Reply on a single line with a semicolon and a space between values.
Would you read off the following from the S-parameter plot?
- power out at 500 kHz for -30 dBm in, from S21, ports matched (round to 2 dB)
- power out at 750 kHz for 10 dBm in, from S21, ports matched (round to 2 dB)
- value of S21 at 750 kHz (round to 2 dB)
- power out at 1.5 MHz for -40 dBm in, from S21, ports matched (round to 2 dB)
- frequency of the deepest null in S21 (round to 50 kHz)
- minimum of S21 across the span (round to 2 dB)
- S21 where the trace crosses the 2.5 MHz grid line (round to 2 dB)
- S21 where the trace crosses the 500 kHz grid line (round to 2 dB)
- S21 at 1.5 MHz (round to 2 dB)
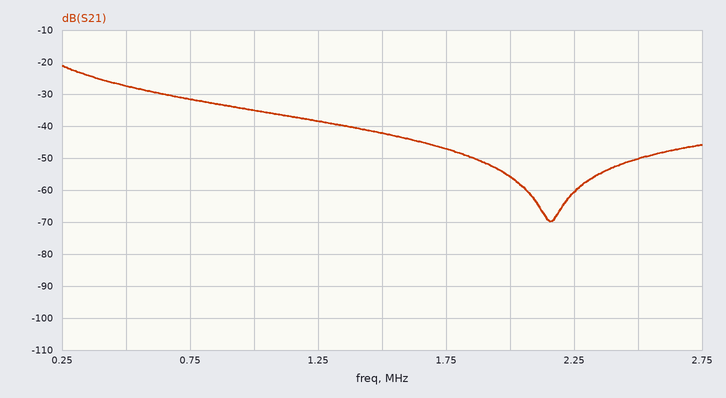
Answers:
-58 dBm; -22 dBm; -32 dB; -82 dBm; 2.15 MHz; -70 dB; -50 dB; -28 dB; -42 dB
